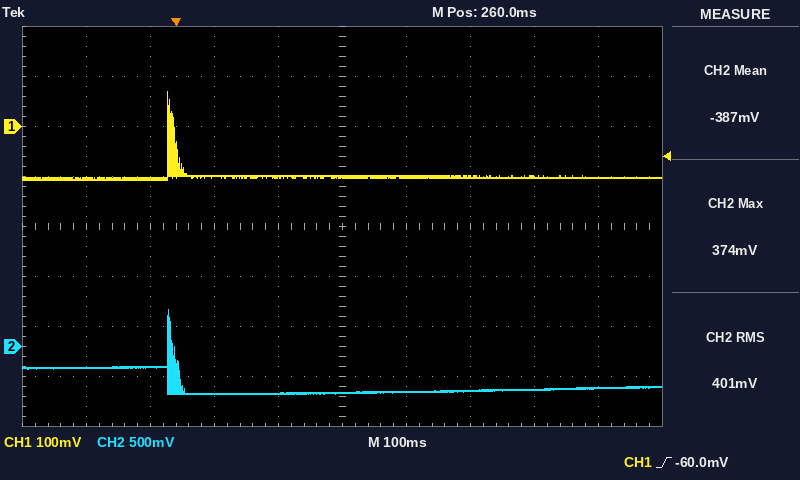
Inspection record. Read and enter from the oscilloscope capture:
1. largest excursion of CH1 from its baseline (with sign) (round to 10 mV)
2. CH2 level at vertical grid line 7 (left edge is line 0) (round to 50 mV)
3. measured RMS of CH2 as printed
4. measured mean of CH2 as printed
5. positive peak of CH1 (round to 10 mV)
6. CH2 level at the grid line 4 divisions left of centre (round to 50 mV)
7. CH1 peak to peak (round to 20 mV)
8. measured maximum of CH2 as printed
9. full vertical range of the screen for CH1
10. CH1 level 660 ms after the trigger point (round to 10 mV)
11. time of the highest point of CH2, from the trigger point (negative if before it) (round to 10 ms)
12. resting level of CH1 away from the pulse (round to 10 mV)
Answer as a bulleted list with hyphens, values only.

- +170 mV
- -450 mV
- 401 mV
- -387 mV
- 70 mV
- -200 mV
- 180 mV
- 374 mV
- 800 mV
- -100 mV
- -10 ms
- -100 mV
